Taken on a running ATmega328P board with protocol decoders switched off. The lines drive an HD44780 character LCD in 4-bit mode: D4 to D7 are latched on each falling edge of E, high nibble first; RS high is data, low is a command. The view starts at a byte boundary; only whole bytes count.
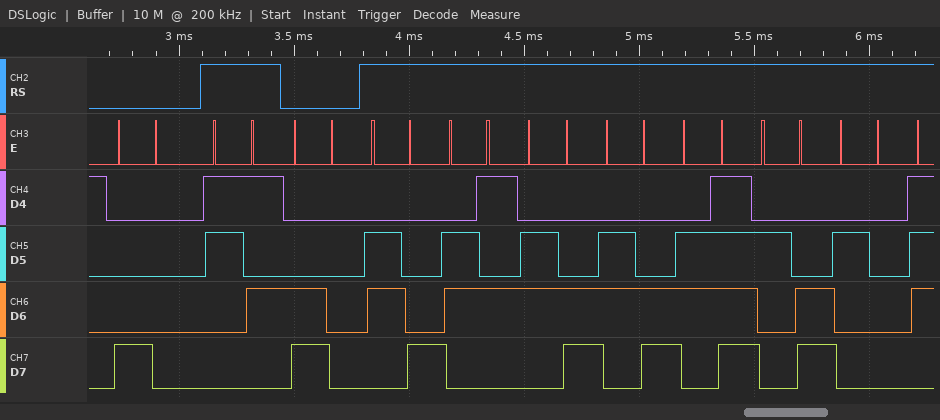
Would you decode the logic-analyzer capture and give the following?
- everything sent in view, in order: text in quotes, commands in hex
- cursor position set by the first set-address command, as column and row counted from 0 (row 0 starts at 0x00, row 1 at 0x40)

0x80 "5" 0xC0 "hello, "
column 0, row 0
